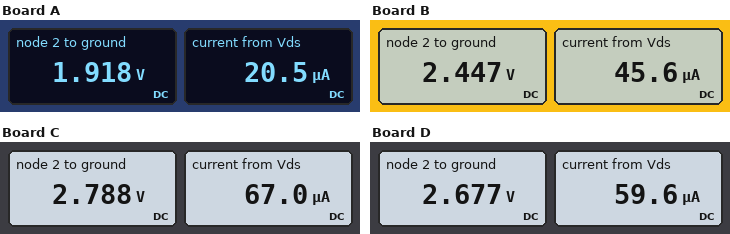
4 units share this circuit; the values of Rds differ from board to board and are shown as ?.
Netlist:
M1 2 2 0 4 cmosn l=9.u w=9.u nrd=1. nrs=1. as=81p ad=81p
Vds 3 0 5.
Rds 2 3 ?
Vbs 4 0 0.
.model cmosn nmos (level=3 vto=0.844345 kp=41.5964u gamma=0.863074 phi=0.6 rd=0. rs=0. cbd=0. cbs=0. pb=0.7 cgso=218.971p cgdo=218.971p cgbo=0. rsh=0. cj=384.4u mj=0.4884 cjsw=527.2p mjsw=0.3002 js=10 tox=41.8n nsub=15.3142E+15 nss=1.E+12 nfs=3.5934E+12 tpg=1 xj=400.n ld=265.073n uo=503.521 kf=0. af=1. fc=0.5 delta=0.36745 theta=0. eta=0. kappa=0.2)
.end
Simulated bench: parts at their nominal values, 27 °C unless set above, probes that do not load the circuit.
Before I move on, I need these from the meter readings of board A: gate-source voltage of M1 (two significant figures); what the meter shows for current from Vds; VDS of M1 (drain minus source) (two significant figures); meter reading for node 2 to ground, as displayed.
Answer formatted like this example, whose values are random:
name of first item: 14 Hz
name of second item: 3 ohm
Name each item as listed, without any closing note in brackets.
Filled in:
gate-source voltage of M1: 1.9 V
what the meter shows for current from Vds: 20.5 µA
VDS of M1 (drain minus source): 1.9 V
meter reading for node 2 to ground, as displayed: 1.918 V
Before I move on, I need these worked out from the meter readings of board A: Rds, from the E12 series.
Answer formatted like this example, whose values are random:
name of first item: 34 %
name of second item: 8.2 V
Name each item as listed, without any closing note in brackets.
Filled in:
Rds, from the E12 series: 150 kΩ
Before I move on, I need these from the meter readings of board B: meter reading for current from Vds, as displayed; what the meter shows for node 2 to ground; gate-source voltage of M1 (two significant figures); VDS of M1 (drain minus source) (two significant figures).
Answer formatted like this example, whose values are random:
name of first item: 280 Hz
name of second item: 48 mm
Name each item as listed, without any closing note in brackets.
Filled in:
meter reading for current from Vds, as displayed: 45.6 µA
what the meter shows for node 2 to ground: 2.447 V
gate-source voltage of M1: 2.4 V
VDS of M1 (drain minus source): 2.4 V
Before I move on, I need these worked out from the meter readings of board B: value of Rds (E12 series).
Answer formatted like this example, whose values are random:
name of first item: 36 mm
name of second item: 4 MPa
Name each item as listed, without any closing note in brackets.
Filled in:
value of Rds: 56 kΩ
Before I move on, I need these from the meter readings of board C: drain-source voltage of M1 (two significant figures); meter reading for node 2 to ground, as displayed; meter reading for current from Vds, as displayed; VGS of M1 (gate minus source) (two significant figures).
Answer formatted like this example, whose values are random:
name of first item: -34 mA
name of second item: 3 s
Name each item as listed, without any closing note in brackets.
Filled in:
drain-source voltage of M1: 2.8 V
meter reading for node 2 to ground, as displayed: 2.788 V
meter reading for current from Vds, as displayed: 67.0 µA
VGS of M1 (gate minus source): 2.8 V
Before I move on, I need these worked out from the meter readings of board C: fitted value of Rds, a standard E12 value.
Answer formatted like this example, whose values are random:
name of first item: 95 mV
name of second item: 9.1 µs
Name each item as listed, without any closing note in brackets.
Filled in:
fitted value of Rds, a standard E12 value: 33 kΩ
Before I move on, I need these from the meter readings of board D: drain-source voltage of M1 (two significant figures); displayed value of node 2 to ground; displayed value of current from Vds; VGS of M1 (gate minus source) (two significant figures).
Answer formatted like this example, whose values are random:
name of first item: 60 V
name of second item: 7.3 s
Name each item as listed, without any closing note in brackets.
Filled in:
drain-source voltage of M1: 2.7 V
displayed value of node 2 to ground: 2.677 V
displayed value of current from Vds: 59.6 µA
VGS of M1 (gate minus source): 2.7 V
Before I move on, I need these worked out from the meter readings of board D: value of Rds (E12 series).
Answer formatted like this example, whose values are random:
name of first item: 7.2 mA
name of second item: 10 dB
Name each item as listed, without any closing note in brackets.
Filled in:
value of Rds: 39 kΩ
